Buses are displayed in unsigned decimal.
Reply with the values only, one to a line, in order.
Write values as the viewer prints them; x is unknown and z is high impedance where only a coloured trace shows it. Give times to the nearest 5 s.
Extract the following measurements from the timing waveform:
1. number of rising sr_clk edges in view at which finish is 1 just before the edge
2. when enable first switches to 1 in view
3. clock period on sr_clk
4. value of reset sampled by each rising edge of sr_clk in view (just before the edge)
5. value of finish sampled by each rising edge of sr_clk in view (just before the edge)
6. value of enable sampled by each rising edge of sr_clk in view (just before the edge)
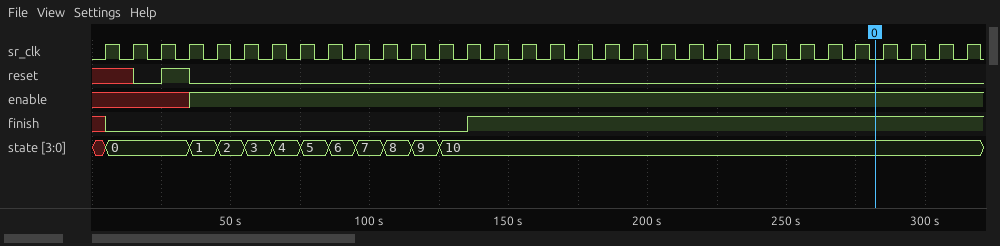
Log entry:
18
35 s
10 s
x x 0 1 0 0 0 0 0 0 0 0 0 0 0 0 0 0 0 0 0 0 0 0 0 0 0 0 0 0 0 0
x 0 0 0 0 0 0 0 0 0 0 0 0 0 1 1 1 1 1 1 1 1 1 1 1 1 1 1 1 1 1 1
x x x x 1 1 1 1 1 1 1 1 1 1 1 1 1 1 1 1 1 1 1 1 1 1 1 1 1 1 1 1
